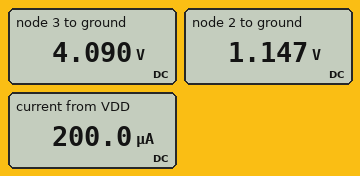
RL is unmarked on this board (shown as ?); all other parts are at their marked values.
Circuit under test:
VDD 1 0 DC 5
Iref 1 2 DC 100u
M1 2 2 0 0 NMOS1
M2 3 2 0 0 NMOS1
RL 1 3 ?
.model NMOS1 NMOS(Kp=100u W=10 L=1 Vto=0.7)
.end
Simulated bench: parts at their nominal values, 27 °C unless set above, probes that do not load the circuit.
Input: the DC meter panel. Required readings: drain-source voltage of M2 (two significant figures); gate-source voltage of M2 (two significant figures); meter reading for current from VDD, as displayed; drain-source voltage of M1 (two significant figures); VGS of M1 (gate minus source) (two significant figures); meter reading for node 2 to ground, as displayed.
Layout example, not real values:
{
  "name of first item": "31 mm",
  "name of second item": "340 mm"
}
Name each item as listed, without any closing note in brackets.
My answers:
{
  "drain-source voltage of M2": "4.1 V",
  "gate-source voltage of M2": "1.1 V",
  "meter reading for current from VDD, as displayed": "200.0 µA",
  "drain-source voltage of M1": "1.1 V",
  "VGS of M1 (gate minus source)": "1.1 V",
  "meter reading for node 2 to ground, as displayed": "1.147 V"
}
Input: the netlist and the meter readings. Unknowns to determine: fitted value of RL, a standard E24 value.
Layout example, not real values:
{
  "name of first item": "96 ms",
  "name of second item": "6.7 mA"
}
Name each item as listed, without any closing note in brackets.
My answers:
{
  "fitted value of RL, a standard E24 value": "9.1 kΩ"
}
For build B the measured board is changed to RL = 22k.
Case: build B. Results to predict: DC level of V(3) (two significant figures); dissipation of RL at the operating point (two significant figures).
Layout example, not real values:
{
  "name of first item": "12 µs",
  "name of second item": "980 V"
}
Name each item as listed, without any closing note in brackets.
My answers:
{
  "DC level of V(3)": "2.8 V",
  "dissipation of RL at the operating point": "220 µW"
}
